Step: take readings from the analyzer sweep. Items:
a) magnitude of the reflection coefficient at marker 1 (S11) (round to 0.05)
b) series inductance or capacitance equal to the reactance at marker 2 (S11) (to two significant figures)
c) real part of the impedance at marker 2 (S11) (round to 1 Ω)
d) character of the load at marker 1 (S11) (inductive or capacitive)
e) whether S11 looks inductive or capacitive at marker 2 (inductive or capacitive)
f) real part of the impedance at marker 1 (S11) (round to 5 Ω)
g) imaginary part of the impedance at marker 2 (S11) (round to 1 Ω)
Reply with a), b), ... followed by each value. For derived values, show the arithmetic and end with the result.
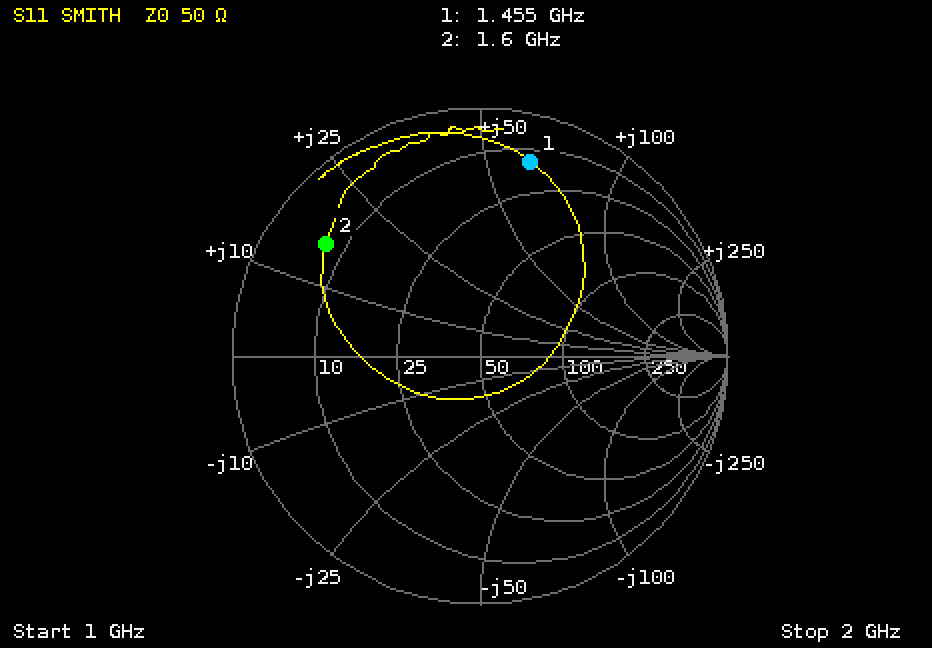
a) 0.80
b) L = 16 Ω/(2π × 1.6 GHz) ≈ 1.6 nH
c) 7 Ω
d) inductive
e) inductive
f) 15 Ω
g) +16 Ω
